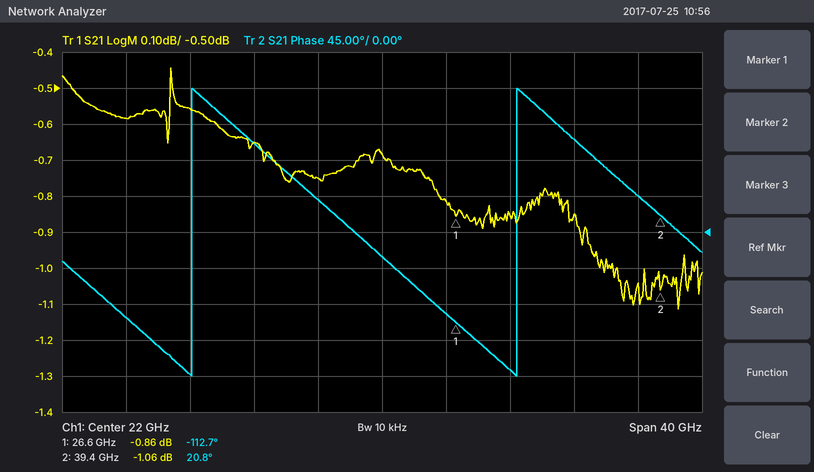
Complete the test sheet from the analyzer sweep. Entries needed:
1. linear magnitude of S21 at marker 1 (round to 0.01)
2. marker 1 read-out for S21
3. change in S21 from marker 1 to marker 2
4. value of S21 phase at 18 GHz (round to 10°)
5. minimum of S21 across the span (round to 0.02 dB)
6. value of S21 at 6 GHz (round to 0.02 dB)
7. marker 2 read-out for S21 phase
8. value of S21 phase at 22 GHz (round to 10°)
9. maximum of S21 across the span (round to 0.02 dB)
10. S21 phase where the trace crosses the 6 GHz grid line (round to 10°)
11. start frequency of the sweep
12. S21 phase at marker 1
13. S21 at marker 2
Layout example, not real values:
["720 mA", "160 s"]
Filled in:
["0.91", "-0.86 dB", "-0.20 dB", "40°", "-1.12 dB", "-0.58 dB", "20.8°", "-30°", "-0.44 dB", "-110°", "2 GHz", "-112.7°", "-1.06 dB"]
